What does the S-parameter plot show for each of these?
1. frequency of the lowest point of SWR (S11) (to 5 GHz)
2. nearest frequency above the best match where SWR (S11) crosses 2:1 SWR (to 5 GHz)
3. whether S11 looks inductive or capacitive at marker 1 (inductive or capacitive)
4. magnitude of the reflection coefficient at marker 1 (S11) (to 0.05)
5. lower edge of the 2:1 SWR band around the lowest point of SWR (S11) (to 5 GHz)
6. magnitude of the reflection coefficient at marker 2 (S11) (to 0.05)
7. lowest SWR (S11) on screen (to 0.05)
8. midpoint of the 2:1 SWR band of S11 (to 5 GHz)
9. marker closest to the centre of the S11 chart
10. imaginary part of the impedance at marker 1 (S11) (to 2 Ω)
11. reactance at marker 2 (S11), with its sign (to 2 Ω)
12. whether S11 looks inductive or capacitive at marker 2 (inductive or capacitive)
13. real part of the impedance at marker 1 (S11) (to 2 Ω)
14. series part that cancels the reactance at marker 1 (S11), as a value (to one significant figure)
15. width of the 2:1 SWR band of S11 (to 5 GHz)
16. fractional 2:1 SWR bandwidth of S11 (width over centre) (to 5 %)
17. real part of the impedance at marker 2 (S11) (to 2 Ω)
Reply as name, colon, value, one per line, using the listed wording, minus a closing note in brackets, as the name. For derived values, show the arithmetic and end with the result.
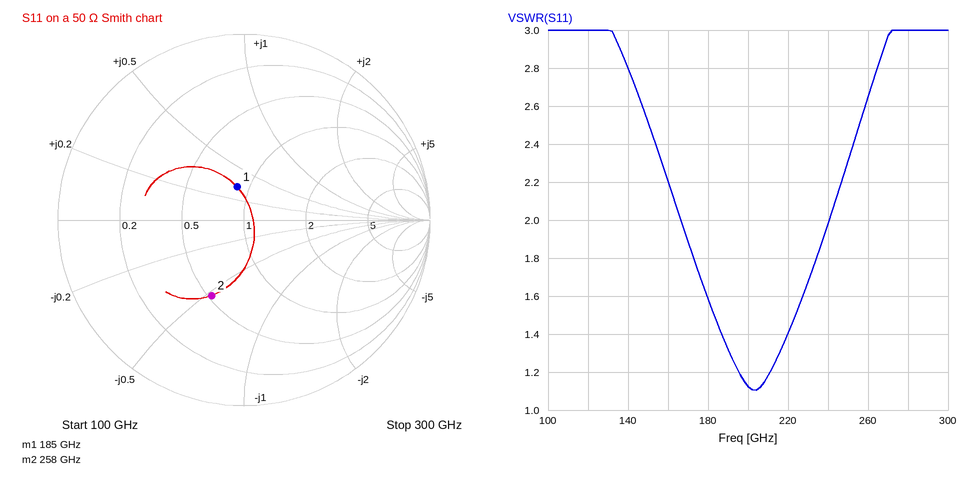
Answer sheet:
frequency of the lowest point of SWR (S11): 205 GHz
nearest frequency above the best match where SWR (S11) crosses 2:1 SWR: 240 GHz
whether S11 looks inductive or capacitive at marker 1: inductive
magnitude of the reflection coefficient at marker 1 (S11): 0.20
lower edge of the 2:1 SWR band around the lowest point of SWR (S11): 165 GHz
magnitude of the reflection coefficient at marker 2 (S11): 0.45
lowest SWR (S11) on screen: 1.10
midpoint of the 2:1 SWR band of S11: 205 GHz
marker closest to the centre of the S11 chart: marker 1
imaginary part of the impedance at marker 1 (S11): +16 Ω
reactance at marker 2 (S11), with its sign: -26 Ω
whether S11 looks inductive or capacitive at marker 2: capacitive
real part of the impedance at marker 1 (S11): 44 Ω
series part that cancels the reactance at marker 1 (S11), as a value: C = 1/(2π × 185 GHz × 16 Ω) ≈ 53.8 fF, so 50 fF to one significant figure
width of the 2:1 SWR band of S11: 240 GHz − 165 GHz = 75 GHz
fractional 2:1 SWR bandwidth of S11 (width over centre): 75 GHz / 202.5 GHz ≈ 37.0 %, so 35 % to the nearest 5 %
real part of the impedance at marker 2 (S11): 26 Ω
